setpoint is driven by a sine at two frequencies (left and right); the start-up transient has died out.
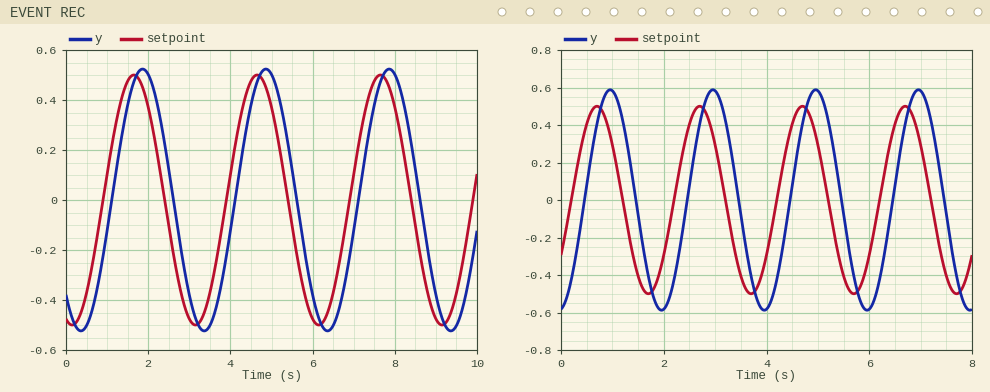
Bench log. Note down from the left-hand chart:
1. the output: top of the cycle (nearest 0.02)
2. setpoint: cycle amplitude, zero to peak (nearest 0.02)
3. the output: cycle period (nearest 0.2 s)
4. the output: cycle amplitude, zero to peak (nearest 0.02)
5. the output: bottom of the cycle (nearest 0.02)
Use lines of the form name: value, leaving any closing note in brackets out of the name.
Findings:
the output: top of the cycle: 0.52
setpoint: cycle amplitude, zero to peak: 0.50
the output: cycle period: 3.0 s
the output: cycle amplitude, zero to peak: 0.52
the output: bottom of the cycle: -0.52
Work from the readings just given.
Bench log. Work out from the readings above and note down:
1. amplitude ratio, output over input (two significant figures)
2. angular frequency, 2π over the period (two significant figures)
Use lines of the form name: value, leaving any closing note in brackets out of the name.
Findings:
amplitude ratio, output over input: 1.0
angular frequency, 2π over the period: 2.1 rad/s
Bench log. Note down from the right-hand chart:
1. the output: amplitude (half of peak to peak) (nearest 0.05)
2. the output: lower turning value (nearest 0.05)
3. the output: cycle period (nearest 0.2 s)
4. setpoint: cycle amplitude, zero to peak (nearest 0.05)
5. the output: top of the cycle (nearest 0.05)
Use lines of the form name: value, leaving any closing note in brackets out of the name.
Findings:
the output: amplitude (half of peak to peak): 0.60
the output: lower turning value: -0.60
the output: cycle period: 2.0 s
setpoint: cycle amplitude, zero to peak: 0.50
the output: top of the cycle: 0.60
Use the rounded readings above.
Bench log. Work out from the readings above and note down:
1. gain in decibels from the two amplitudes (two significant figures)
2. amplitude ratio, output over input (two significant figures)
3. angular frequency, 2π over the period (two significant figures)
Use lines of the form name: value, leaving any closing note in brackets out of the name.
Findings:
gain in decibels from the two amplitudes: 1.6 dB
amplitude ratio, output over input: 1.2
angular frequency, 2π over the period: 3.1 rad/s
